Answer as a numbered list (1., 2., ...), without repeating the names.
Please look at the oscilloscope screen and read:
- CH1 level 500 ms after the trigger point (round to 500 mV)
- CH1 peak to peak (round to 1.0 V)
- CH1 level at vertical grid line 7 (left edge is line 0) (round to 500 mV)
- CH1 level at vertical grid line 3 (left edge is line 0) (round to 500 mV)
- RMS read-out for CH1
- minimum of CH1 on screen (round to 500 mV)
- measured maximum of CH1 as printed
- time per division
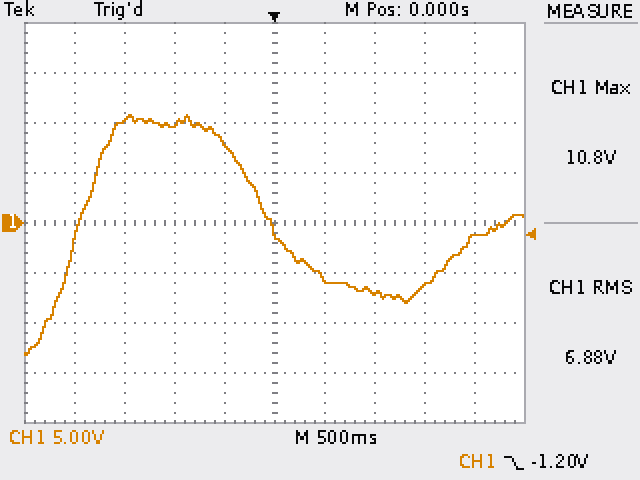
1. -5.5 V
2. 24.0 V
3. -7.0 V
4. 10.0 V
5. 6.88 V
6. -13.0 V
7. 10.8 V
8. 500 ms
